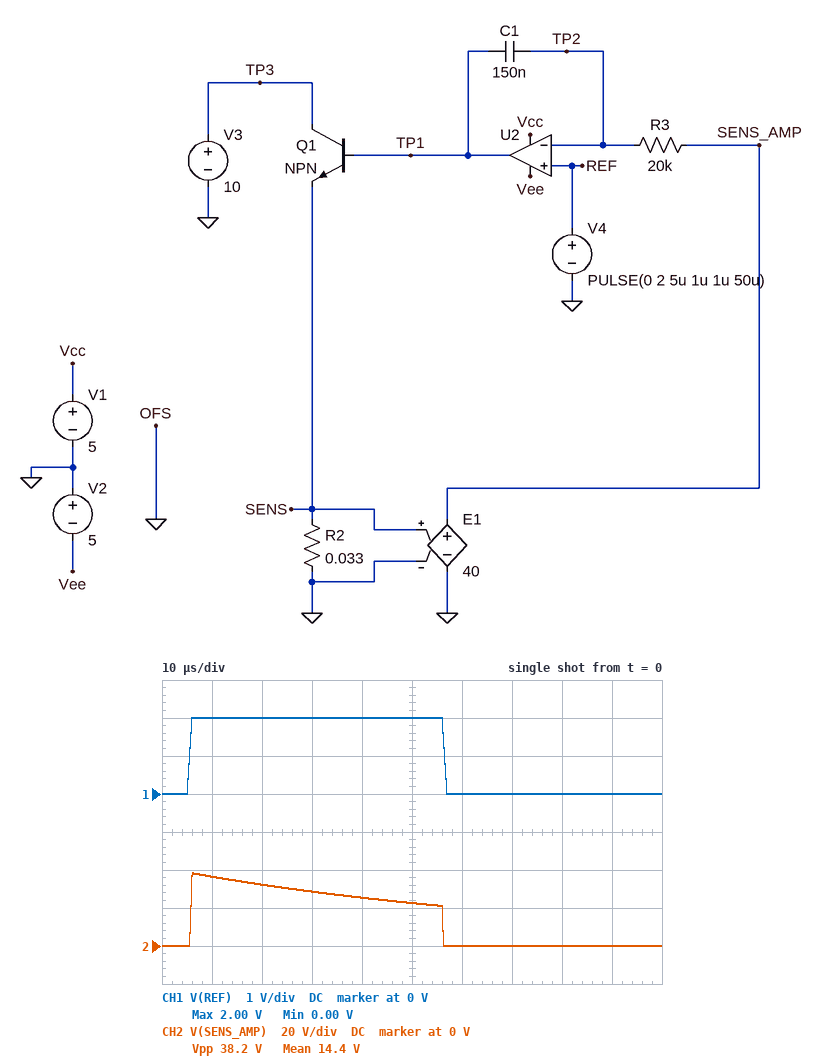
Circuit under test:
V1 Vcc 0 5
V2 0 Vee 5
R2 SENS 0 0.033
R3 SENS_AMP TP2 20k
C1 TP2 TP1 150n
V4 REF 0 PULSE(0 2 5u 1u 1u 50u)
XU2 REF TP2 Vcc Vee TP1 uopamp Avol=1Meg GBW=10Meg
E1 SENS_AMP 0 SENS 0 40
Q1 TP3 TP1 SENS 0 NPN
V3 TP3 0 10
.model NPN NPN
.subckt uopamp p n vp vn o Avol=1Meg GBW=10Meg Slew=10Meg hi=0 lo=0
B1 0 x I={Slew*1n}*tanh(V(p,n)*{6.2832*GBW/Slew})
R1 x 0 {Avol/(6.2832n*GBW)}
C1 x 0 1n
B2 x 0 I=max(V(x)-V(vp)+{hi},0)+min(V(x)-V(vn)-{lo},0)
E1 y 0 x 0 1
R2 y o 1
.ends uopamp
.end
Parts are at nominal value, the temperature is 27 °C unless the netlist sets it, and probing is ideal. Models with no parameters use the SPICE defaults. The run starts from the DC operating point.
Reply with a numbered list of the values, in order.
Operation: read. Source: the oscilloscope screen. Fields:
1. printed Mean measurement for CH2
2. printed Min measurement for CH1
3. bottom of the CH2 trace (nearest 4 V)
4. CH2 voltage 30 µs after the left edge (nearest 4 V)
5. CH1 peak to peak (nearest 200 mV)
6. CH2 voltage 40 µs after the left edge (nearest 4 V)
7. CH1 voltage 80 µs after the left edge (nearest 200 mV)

1. 14.4 V
2. 0.00 V
3. 0 V
4. 28 V
5. 2.0 V
6. 24 V
7. 0 V
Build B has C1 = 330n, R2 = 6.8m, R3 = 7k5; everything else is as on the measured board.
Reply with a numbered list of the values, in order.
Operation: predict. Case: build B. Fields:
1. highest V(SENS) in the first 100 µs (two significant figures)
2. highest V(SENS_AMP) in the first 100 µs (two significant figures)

1. 920 mV
2. 37 V
